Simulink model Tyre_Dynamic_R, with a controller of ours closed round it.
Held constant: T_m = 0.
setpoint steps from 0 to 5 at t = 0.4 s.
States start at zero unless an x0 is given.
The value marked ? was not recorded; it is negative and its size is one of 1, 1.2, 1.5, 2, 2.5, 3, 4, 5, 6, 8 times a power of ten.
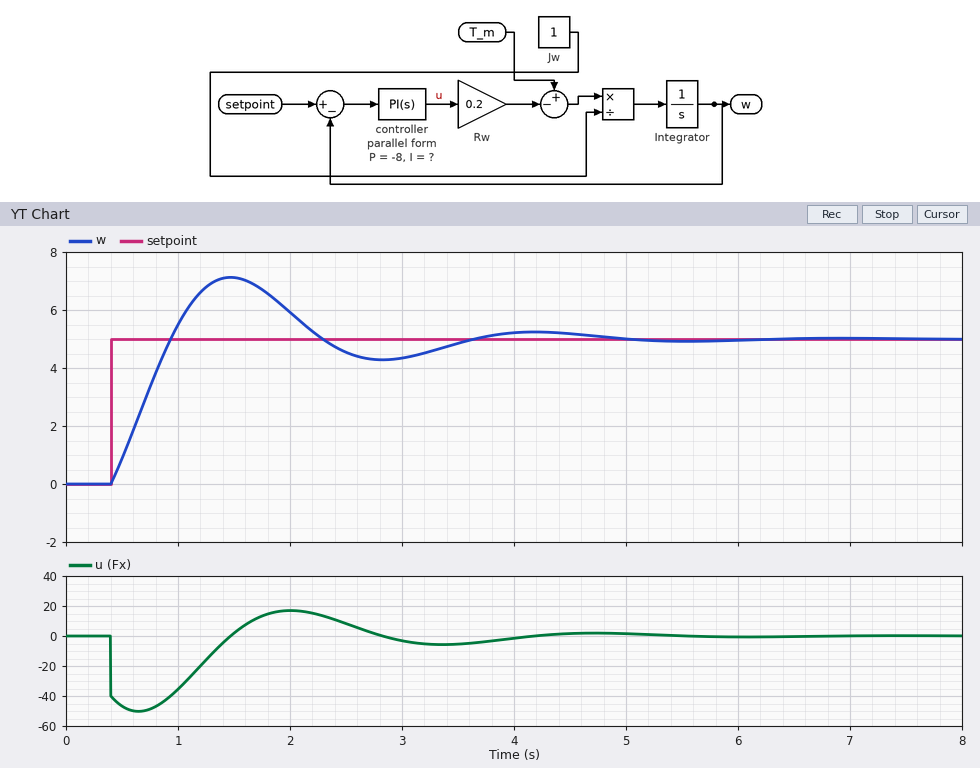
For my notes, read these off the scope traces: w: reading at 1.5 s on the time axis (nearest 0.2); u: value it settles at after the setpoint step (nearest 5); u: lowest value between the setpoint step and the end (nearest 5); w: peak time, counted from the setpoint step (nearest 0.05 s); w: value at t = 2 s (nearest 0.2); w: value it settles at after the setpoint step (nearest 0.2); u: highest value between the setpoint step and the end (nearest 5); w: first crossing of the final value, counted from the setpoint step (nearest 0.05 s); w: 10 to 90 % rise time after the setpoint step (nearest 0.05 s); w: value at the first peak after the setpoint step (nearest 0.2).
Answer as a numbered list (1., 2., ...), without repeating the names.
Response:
1. 7.2
2. 0
3. -50
4. 1.05 s
5. 6.0
6. 5.0
7. 15
8. 0.55 s
9. 0.40 s
10. 7.2
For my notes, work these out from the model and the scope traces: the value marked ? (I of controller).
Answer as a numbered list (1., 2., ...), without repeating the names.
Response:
1. -30
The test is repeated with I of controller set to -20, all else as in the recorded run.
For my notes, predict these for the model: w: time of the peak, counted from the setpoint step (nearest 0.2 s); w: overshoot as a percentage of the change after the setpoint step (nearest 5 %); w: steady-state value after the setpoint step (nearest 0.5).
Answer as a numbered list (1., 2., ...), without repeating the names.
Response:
1. 1.2 s
2. 35 %
3. 5.0
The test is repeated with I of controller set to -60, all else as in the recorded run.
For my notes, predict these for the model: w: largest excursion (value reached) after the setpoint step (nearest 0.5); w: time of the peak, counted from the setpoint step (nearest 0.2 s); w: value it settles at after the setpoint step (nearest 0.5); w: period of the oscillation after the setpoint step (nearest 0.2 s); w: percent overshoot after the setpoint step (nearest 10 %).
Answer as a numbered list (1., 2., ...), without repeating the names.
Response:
1. 7.5
2. 0.8 s
3. 5.0
4. 1.8 s
5. 50 %
